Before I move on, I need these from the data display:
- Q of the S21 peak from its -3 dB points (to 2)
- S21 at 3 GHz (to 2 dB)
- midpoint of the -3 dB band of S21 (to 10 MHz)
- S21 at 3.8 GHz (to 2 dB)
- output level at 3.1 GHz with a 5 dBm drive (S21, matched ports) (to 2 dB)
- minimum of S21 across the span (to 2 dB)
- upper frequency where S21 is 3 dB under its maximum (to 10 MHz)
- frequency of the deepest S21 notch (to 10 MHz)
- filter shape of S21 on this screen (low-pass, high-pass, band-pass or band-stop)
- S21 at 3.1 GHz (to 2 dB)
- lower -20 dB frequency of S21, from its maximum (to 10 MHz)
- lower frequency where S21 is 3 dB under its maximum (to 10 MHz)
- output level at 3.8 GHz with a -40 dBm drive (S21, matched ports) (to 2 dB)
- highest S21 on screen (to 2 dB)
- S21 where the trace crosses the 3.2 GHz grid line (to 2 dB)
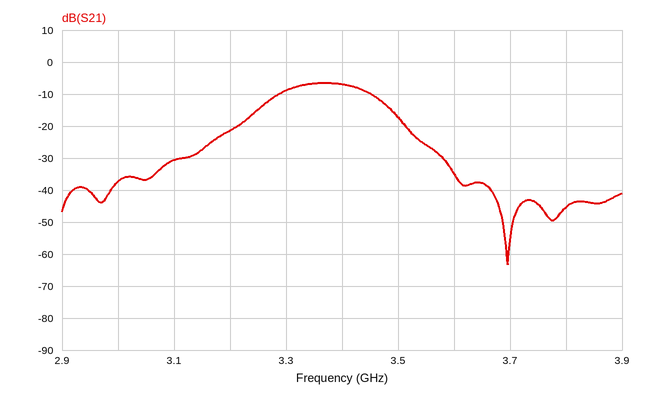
22
-38 dB
3.37 GHz
-46 dB
-26 dBm
-64 dB
3.45 GHz
3.70 GHz
band-pass
-30 dB
3.16 GHz
3.29 GHz
-86 dBm
-6 dB
-22 dB
